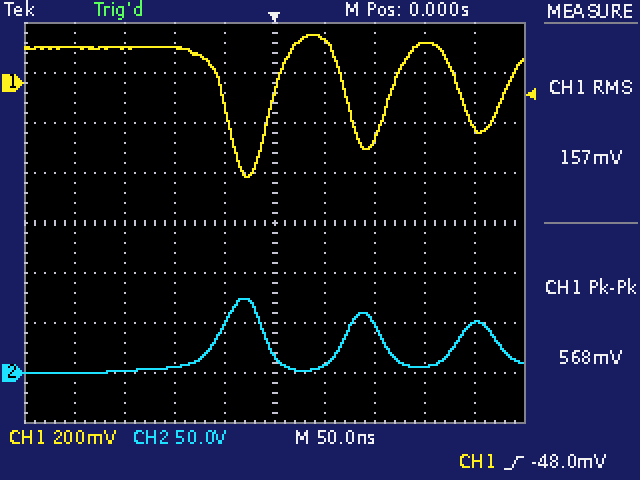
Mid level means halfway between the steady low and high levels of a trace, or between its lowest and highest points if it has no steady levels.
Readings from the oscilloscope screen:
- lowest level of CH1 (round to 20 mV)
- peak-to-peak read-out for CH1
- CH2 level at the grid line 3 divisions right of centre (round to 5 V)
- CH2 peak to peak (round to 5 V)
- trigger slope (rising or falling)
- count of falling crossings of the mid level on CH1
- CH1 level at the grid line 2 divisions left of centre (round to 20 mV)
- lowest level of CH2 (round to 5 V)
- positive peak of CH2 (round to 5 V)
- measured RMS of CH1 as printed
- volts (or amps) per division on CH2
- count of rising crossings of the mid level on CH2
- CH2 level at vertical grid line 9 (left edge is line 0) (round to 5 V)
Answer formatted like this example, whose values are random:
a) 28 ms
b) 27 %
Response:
a) -380 mV
b) 568 mV
c) 5 V
d) 75 V
e) rising
f) 3
g) 140 mV
h) 0 V
i) 75 V
j) 157 mV
k) 50 V
l) 3
m) 50 V
